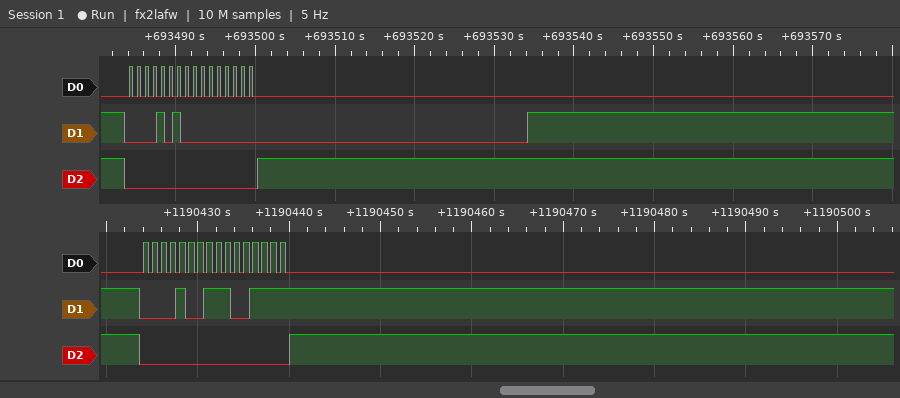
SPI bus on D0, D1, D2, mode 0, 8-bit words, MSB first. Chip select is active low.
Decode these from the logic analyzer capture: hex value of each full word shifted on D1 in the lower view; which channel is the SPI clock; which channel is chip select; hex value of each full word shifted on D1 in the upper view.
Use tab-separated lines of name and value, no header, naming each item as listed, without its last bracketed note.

hex value of each full word shifted on D1 in the lower view	09, CF
which channel is the SPI clock	D0
which channel is chip select	D2
hex value of each full word shifted on D1 in the upper view	0A, 00
